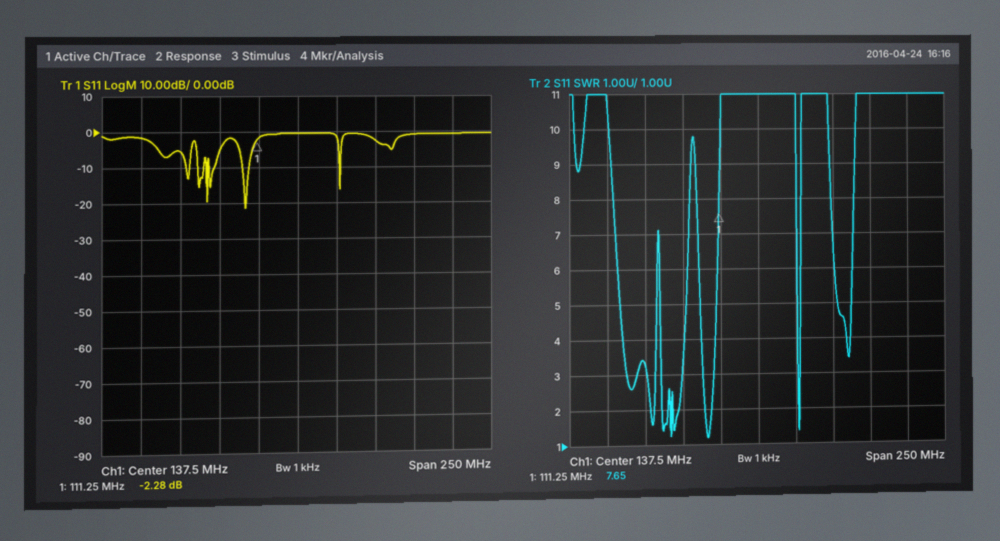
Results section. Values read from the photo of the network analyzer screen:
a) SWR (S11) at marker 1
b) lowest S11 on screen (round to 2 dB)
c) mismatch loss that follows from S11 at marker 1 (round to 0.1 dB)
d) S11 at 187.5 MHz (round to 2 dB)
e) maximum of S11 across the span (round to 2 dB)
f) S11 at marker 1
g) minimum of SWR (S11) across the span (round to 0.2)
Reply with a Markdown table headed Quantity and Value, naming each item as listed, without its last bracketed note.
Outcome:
| Quantity | Value |
|---|---|
| SWR (S11) at marker 1 | 7.65 |
| lowest S11 on screen | -22 dB |
| mismatch loss that follows from S11 at marker 1 | 3.9 dB |
| S11 at 187.5 MHz | -2 dB |
| maximum of S11 across the span | 0 dB |
| S11 at marker 1 | -2.28 dB |
| minimum of SWR (S11) across the span | 1.2 |
